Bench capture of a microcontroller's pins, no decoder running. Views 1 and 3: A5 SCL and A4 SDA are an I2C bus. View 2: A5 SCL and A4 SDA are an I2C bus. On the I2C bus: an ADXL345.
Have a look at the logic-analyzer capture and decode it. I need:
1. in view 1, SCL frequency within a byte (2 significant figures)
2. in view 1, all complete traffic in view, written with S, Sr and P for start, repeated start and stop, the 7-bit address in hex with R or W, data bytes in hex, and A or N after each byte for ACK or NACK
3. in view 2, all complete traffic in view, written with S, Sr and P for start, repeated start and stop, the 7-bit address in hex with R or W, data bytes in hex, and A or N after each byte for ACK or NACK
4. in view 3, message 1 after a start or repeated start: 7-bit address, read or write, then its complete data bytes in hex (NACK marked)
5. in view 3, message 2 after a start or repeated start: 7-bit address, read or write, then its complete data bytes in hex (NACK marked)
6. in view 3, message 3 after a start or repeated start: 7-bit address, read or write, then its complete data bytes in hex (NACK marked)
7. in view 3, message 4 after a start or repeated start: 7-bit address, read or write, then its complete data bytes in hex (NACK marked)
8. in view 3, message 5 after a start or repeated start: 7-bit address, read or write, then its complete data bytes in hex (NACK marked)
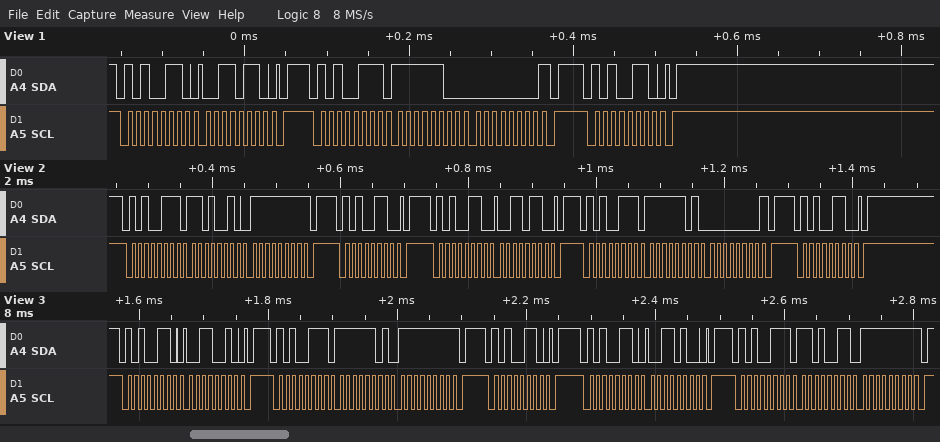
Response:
100 kHz
S 53W A 36 A P S 53R A FC A 00 N P S 53W A P
S 53R A D2 A FF N P S 53W A P S 53W A 36 A P S 53R A FD A 00 N P S 53W A P
0x53 write: 32
0x53 read: FD FF NACK
0x53 write
0x53 write: 34
0x53 read: D3 FF NACK
